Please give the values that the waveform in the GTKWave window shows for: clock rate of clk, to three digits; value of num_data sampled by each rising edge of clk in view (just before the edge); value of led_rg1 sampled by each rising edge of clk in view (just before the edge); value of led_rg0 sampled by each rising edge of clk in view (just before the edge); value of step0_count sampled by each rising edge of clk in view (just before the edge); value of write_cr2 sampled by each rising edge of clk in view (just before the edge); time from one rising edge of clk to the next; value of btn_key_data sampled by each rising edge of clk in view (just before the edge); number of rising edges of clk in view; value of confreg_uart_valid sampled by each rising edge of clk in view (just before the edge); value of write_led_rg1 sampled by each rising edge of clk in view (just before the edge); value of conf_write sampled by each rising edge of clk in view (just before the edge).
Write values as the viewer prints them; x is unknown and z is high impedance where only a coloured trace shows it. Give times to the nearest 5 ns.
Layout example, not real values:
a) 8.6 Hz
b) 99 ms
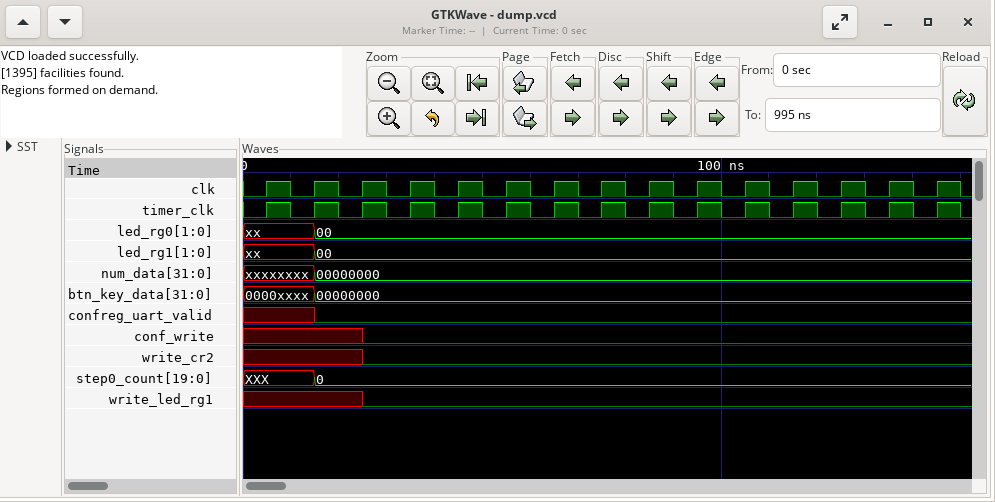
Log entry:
a) 100 MHz
b) xxxxxxxx, xxxxxxxx, 00000000, 00000000, 00000000, 00000000, 00000000, 00000000, 00000000, 00000000, 00000000, 00000000, 00000000, 00000000, 00000000
c) xx, xx, 00, 00, 00, 00, 00, 00, 00, 00, 00, 00, 00, 00, 00
d) xx, xx, 00, 00, 00, 00, 00, 00, 00, 00, 00, 00, 00, 00, 00
e) XXX, XXX, 0, 0, 0, 0, 0, 0, 0, 0, 0, 0, 0, 0, 0
f) x x x 0 0 0 0 0 0 0 0 0 0 0 0
g) 10 ns
h) 0000xxxx, 0000xxxx, 00000000, 00000000, 00000000, 00000000, 00000000, 00000000, 00000000, 00000000, 00000000, 00000000, 00000000, 00000000, 00000000
i) 15
j) x x 0 0 0 0 0 0 0 0 0 0 0 0 0
k) x x x 0 0 0 0 0 0 0 0 0 0 0 0
l) x x x 0 0 0 0 0 0 0 0 0 0 0 0
